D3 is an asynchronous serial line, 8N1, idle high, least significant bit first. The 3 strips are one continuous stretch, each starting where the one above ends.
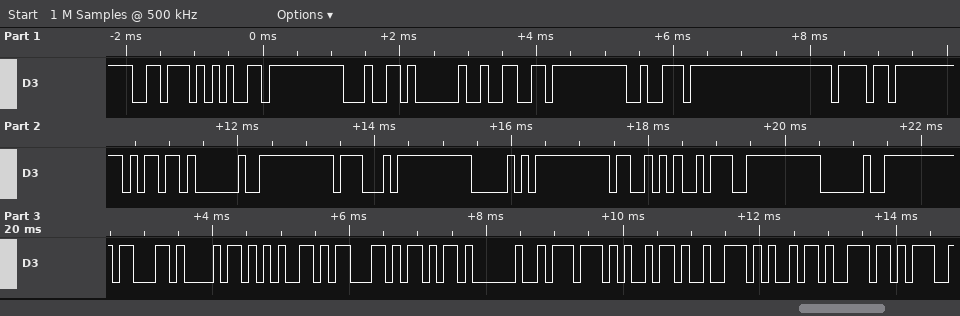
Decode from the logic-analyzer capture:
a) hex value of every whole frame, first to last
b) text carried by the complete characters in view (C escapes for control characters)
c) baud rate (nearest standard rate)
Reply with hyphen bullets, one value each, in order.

- 76 65 64 20 66 72 6F 6D 20 47 50 53 3A 20 63 68 65 63 6B 20 77 69 72 69 6E
- "ved from GPS: check wirin"
- 9600 baud
